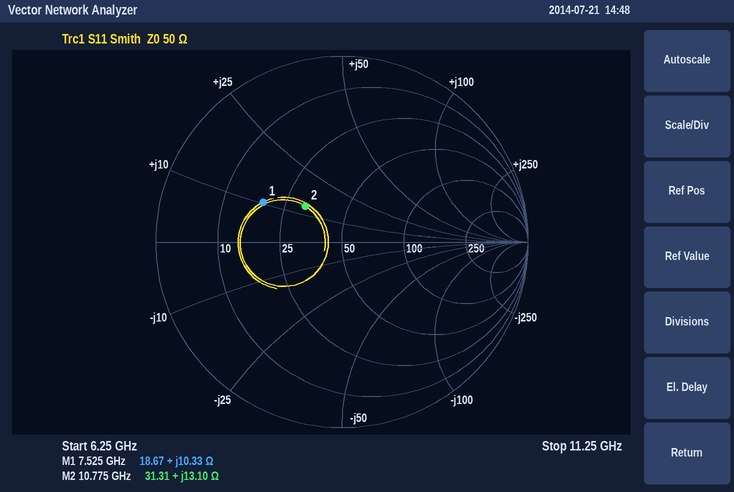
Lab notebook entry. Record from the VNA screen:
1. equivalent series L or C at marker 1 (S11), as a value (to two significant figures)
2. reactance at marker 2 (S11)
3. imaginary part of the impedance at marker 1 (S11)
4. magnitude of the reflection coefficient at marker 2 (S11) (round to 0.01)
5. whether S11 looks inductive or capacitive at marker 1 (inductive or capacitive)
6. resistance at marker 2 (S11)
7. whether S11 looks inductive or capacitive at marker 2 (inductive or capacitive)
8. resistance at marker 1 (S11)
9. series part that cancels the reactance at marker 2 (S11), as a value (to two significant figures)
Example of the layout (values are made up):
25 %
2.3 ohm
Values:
220 pH
+13.10 Ω
+10.33 Ω
0.28
inductive
31.31 Ω
inductive
18.67 Ω
1.1 pF
